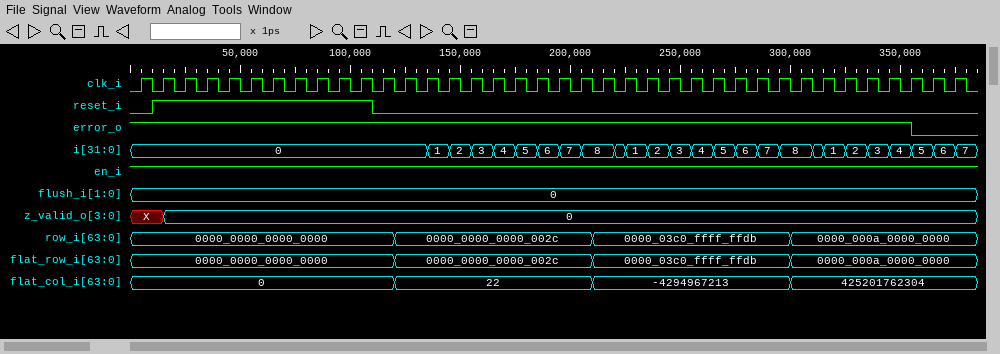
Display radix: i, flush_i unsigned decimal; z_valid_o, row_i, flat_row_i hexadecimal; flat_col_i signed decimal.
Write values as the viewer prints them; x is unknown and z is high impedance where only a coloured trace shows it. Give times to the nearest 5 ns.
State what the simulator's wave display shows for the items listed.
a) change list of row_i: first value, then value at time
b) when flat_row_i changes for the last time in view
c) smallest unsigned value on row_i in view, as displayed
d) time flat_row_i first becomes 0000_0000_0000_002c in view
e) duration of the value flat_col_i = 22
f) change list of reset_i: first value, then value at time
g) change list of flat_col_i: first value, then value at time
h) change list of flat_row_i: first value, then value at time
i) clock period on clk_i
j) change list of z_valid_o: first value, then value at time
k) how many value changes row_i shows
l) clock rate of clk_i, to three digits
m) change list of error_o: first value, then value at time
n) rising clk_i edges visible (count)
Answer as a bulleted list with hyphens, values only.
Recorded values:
- 0000_0000_0000_0000, 0000_0000_0000_002c at 120 ns, 0000_03c0_ffff_ffdb at 210 ns, 0000_000a_0000_0000 at 300 ns
- 300 ns
- 0000_0000_0000_0000
- 120 ns
- 90 ns
- 0, 1 at 10 ns, 0 at 110 ns
- 0, 22 at 120 ns, -4294967213 at 210 ns, 425201762304 at 300 ns
- 0000_0000_0000_0000, 0000_0000_0000_002c at 120 ns, 0000_03c0_ffff_ffdb at 210 ns, 0000_000a_0000_0000 at 300 ns
- 10 ns
- X, 0 at 15 ns
- 3
- 100 MHz
- 1, 0 at 355 ns
- 38
